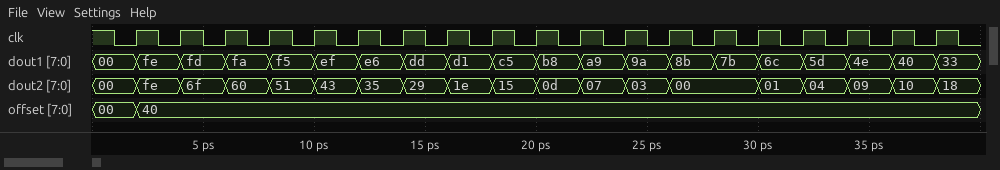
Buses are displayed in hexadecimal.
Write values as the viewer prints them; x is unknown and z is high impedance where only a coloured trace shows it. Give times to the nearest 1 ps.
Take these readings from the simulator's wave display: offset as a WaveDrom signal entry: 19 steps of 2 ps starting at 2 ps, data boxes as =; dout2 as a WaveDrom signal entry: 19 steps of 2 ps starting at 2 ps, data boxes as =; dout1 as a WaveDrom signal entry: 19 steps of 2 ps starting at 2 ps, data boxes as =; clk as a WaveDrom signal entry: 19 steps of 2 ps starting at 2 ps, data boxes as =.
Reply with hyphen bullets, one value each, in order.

- {name: 'offset', wave: '=..................', data: '40'}
- {name: 'dout2', wave: '=============.=====', data: 'fe 6f 60 51 43 35 29 1e 15 0d 07 03 00 01 04 09 10 18'}
- {name: 'dout1', wave: '===================', data: 'fe fd fa f5 ef e6 dd d1 c5 b8 a9 9a 8b 7b 6c 5d 4e 40 33'}
- {name: 'clk', wave: 'p..................'}
